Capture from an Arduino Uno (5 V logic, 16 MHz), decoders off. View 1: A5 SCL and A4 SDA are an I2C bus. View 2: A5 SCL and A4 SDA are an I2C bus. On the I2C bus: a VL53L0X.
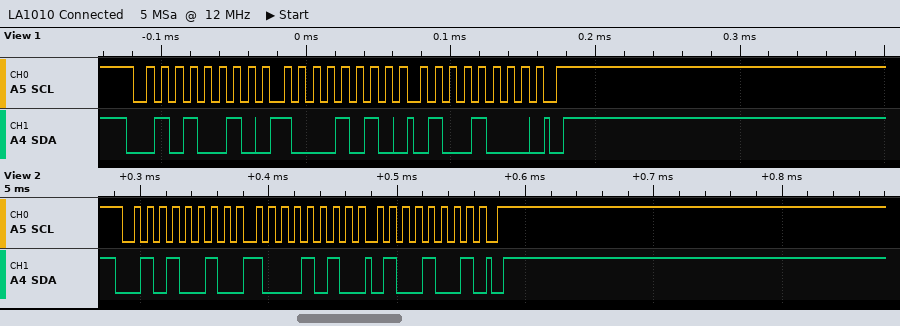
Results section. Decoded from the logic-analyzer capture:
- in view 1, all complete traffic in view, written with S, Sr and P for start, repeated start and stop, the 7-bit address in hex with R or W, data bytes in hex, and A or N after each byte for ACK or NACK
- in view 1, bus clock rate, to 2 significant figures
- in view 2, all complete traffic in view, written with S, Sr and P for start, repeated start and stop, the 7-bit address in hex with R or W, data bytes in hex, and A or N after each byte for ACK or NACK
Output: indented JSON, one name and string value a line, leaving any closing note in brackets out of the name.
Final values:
{
  "in view 1, all complete traffic in view, written with S, Sr and P for start, repeated start and stop, the 7-bit address in hex with R or W, data bytes in hex, and A or N after each byte for ACK or NACK": "S 29W A 8A A 48 A P",
  "in view 1, bus clock rate, to 2 significant figures": "100 kHz",
  "in view 2, all complete traffic in view, written with S, Sr and P for start, repeated start and stop, the 7-bit address in hex with R or W, data bytes in hex, and A or N after each byte for ACK or NACK": "S 29W A 8A A 49 A P"
}
